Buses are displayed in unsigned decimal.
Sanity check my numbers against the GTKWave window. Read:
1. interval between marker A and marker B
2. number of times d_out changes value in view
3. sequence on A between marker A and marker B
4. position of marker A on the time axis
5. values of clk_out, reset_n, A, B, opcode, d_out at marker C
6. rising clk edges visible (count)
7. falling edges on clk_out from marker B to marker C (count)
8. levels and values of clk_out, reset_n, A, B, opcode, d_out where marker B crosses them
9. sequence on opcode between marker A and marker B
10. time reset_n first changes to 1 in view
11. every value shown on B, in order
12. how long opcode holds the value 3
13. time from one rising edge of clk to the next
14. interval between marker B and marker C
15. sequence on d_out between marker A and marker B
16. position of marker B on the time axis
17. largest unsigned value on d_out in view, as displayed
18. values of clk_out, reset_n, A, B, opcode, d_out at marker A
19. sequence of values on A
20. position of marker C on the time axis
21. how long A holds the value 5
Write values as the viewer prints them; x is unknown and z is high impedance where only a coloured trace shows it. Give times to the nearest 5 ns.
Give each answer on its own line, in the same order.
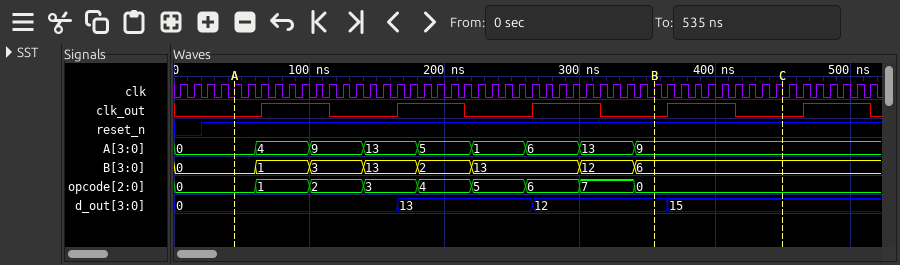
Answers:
310 ns
3
0, 4, 9, 13, 5, 1, 6, 13, 9
45 ns
clk_out=0, reset_n=1, A=9, B=6, opcode=0, d_out=15
52
1
clk_out=0, reset_n=1, A=9, B=6, opcode=0, d_out=12
0, 1, 2, 3, 4, 5, 6, 7, 0
20 ns
0, 1, 3, 13, 2, 13, 12, 6
40 ns
10 ns
95 ns
0, 13, 12
355 ns
15
clk_out=0, reset_n=1, A=0, B=0, opcode=0, d_out=0
0, 4, 9, 13, 5, 1, 6, 13, 9
450 ns
40 ns
